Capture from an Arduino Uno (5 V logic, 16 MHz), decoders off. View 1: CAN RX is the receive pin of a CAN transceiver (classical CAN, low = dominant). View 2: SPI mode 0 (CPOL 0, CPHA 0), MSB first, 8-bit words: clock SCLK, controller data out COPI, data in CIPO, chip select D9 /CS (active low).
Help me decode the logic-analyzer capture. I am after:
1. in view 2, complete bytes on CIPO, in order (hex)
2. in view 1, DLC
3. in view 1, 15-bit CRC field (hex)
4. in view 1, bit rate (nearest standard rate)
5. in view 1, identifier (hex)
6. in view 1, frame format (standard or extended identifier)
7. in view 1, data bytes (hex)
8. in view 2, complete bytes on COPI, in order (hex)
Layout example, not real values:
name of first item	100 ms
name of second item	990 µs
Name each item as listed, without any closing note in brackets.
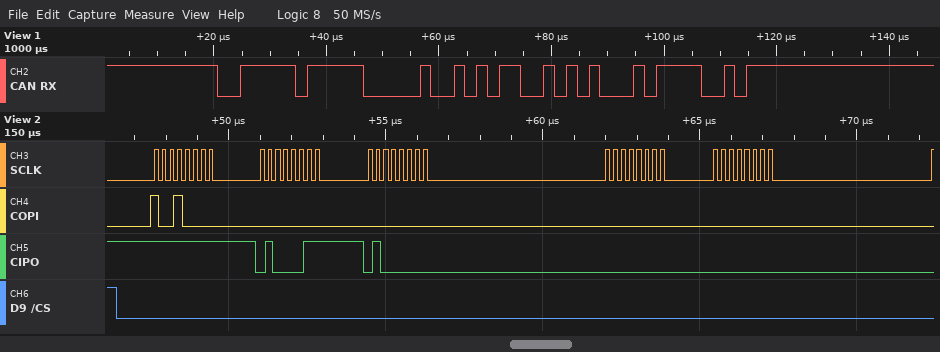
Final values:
in view 2, complete bytes on CIPO, in order	FF 43 40 00 00
in view 1, DLC	1
in view 1, 15-bit CRC field	0x28BC
in view 1, bit rate	500 kbit/s
in view 1, identifier	0x3FF
in view 1, frame format	standard
in view 1, data bytes	59
in view 2, complete bytes on COPI, in order	90 00 00 00 00
